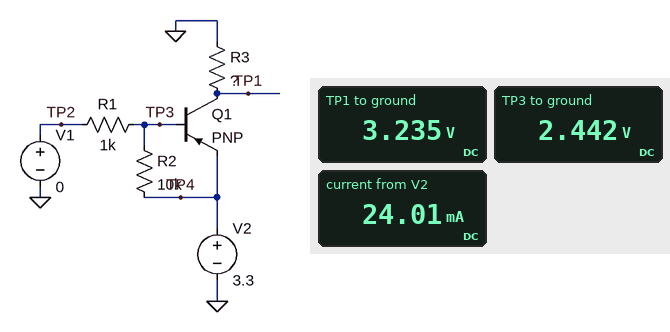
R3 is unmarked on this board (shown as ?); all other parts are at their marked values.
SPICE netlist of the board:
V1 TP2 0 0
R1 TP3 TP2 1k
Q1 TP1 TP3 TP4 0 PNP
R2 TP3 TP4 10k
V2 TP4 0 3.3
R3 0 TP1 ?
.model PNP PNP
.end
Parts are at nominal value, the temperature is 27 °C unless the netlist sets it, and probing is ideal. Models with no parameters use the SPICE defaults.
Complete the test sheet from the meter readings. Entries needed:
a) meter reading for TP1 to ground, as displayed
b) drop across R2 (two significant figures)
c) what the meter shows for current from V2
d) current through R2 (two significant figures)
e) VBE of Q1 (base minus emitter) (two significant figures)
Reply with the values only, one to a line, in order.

3.235 V
860 mV
24.01 mA
86 µA
-860 mV
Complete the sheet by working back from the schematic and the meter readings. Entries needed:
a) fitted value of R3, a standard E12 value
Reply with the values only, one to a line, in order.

150 Ω
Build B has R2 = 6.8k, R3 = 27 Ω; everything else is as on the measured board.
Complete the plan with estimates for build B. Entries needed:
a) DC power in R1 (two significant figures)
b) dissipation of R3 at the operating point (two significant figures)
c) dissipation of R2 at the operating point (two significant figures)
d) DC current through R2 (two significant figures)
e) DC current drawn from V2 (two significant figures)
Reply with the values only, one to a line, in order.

5.8 mW
370 mW
120 µW
130 µA
120 mA
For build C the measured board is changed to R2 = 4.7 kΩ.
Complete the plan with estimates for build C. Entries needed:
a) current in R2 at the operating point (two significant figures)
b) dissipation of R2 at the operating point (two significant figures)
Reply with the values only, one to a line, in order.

180 µA
160 µW
